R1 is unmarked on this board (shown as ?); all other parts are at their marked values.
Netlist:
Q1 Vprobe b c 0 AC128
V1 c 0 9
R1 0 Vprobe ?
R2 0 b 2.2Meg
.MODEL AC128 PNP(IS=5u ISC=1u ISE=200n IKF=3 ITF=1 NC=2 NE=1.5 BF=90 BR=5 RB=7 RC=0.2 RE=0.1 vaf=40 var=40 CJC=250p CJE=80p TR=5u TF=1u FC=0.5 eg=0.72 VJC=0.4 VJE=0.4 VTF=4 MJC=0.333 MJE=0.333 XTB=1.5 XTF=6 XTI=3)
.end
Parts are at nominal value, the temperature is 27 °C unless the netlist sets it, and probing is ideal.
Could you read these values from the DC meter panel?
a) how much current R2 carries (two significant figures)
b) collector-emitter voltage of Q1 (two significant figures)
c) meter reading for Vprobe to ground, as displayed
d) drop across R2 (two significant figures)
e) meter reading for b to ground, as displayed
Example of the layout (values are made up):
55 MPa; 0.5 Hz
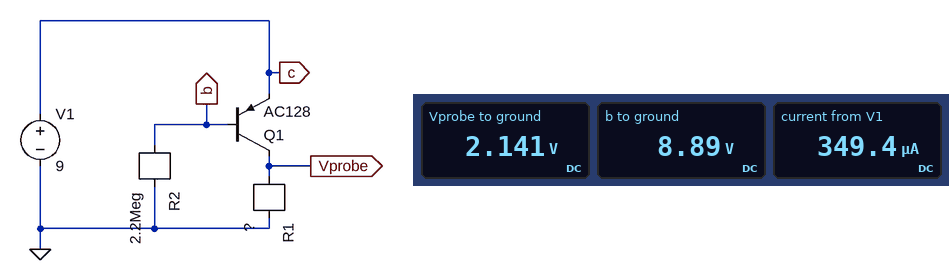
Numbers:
4.0 µA; -6.9 V; 2.141 V; 8.9 V; 8.89 V
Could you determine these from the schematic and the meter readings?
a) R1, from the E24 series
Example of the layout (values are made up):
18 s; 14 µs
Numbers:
6.2 kΩ
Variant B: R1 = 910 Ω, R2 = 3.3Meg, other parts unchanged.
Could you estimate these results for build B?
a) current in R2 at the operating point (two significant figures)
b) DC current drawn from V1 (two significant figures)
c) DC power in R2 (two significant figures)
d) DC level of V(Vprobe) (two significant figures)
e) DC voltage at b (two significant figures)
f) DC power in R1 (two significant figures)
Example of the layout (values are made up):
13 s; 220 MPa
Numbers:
2.7 µA; 270 µA; 24 µW; 250 mV; 8.9 V; 66 µW
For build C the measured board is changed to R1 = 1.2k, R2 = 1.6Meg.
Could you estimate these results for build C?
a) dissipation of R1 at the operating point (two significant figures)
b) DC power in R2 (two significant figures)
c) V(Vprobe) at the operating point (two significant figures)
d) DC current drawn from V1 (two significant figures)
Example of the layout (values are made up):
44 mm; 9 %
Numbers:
250 µW; 49 µW; 550 mV; 470 µA
